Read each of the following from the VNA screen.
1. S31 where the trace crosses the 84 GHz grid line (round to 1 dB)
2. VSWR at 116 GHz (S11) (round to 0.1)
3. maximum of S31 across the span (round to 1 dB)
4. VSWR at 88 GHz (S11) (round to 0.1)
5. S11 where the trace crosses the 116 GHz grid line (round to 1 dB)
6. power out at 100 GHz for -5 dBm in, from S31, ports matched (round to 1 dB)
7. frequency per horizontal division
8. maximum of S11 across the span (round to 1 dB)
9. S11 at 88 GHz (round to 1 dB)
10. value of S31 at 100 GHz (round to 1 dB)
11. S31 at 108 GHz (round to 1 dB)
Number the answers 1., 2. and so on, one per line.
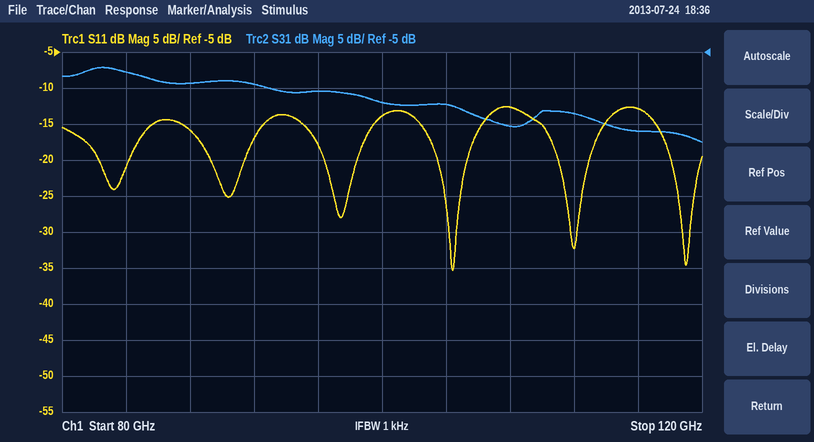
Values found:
1. -8 dB
2. 1.6
3. -7 dB
4. 1.4
5. -13 dB
6. -17 dBm
7. 4 GHz
8. -13 dB
9. -16 dB
10. -12 dB
11. -15 dB
